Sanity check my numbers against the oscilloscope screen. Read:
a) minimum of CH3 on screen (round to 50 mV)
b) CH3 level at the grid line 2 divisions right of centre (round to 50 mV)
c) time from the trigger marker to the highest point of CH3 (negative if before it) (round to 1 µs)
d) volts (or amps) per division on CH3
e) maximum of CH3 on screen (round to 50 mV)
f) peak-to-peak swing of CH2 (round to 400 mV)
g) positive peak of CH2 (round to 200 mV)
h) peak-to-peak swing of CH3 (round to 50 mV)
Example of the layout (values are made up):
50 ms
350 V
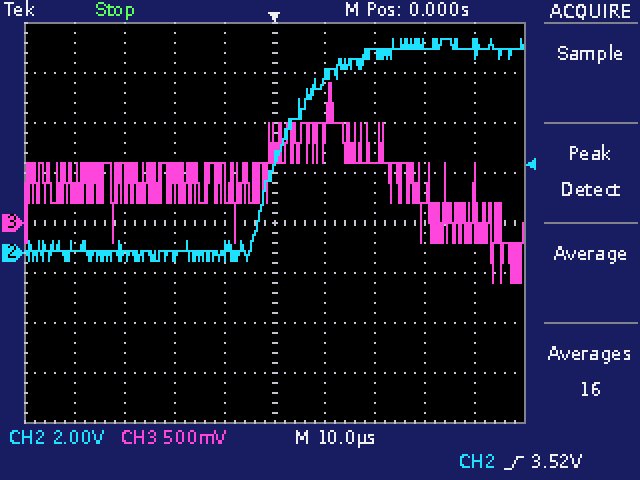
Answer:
-600 mV
600 mV
+11 µs
500 mV
1.40 V
8.8 V
8.6 V
2.00 V
